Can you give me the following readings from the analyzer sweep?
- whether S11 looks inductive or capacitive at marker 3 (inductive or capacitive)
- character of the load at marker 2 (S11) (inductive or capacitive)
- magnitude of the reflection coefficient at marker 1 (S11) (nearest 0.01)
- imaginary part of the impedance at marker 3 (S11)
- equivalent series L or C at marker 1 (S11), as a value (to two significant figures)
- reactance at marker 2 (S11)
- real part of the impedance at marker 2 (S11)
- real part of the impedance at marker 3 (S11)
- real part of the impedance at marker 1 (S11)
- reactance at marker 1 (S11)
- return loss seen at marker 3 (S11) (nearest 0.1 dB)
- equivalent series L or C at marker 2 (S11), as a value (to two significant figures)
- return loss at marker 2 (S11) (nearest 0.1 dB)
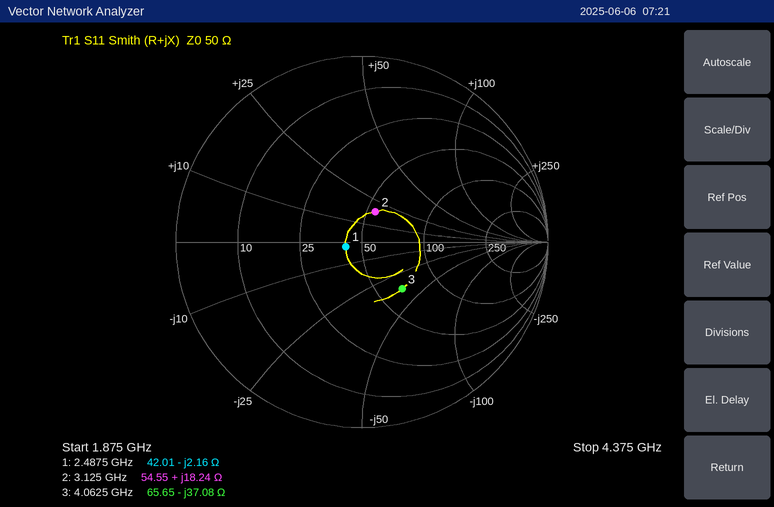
capacitive
inductive
0.09
-37.08 Ω
30 pF
+18.24 Ω
54.55 Ω
65.65 Ω
42.01 Ω
-2.16 Ω
9.6 dB
930 pH
15.0 dB
